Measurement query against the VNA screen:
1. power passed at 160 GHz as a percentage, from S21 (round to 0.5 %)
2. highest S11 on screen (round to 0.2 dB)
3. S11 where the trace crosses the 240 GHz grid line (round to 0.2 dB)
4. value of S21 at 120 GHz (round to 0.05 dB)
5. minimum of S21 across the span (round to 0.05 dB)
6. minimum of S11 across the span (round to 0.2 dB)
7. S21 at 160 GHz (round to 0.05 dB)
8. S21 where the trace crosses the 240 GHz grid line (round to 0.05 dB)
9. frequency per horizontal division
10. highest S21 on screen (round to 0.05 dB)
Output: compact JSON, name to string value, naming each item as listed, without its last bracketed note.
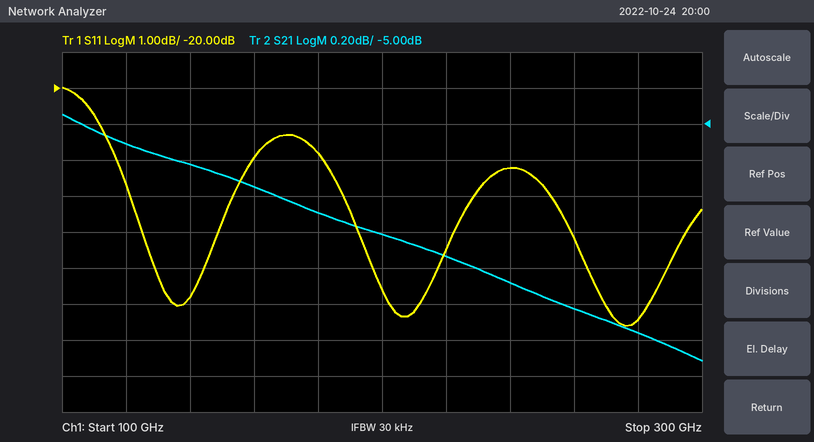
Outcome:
{"power passed at 160 GHz as a percentage, from S21": "29.0 %", "highest S11 on screen": "-20.0 dB", "S11 where the trace crosses the 240 GHz grid line": "-22.2 dB", "value of S21 at 120 GHz": "-5.10 dB", "minimum of S21 across the span": "-6.30 dB", "minimum of S11 across the span": "-26.6 dB", "S21 at 160 GHz": "-5.35 dB", "S21 where the trace crosses the 240 GHz grid line": "-5.90 dB", "frequency per horizontal division": "20 GHz", "highest S21 on screen": "-4.95 dB"}
